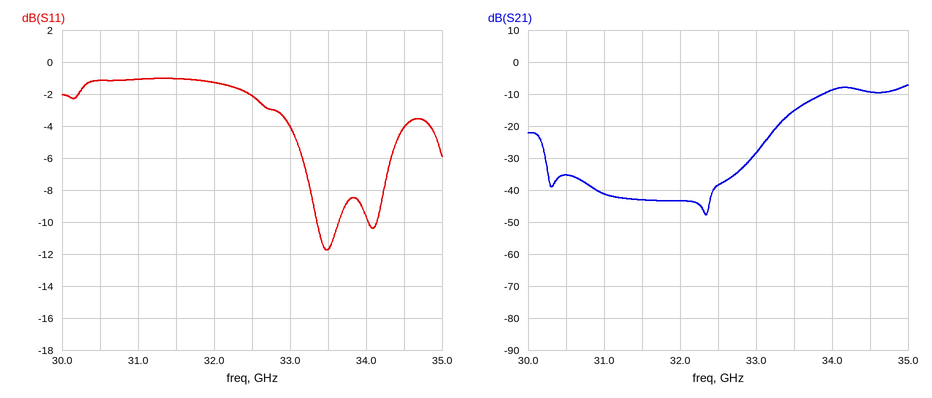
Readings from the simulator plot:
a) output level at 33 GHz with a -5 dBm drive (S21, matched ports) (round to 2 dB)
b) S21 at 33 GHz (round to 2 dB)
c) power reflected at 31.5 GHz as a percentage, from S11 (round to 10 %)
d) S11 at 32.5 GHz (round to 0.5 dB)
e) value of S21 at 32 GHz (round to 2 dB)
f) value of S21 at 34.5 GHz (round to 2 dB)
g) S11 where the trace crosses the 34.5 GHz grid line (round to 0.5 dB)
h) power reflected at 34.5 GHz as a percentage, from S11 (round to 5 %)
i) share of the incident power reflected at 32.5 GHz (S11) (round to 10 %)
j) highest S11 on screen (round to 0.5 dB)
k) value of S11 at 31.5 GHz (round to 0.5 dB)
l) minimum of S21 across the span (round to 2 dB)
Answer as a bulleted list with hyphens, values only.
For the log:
- -34 dBm
- -28 dB
- 80 %
- -2.0 dB
- -44 dB
- -10 dB
- -4.0 dB
- 40 %
- 60 %
- -1.0 dB
- -1.0 dB
- -48 dB
